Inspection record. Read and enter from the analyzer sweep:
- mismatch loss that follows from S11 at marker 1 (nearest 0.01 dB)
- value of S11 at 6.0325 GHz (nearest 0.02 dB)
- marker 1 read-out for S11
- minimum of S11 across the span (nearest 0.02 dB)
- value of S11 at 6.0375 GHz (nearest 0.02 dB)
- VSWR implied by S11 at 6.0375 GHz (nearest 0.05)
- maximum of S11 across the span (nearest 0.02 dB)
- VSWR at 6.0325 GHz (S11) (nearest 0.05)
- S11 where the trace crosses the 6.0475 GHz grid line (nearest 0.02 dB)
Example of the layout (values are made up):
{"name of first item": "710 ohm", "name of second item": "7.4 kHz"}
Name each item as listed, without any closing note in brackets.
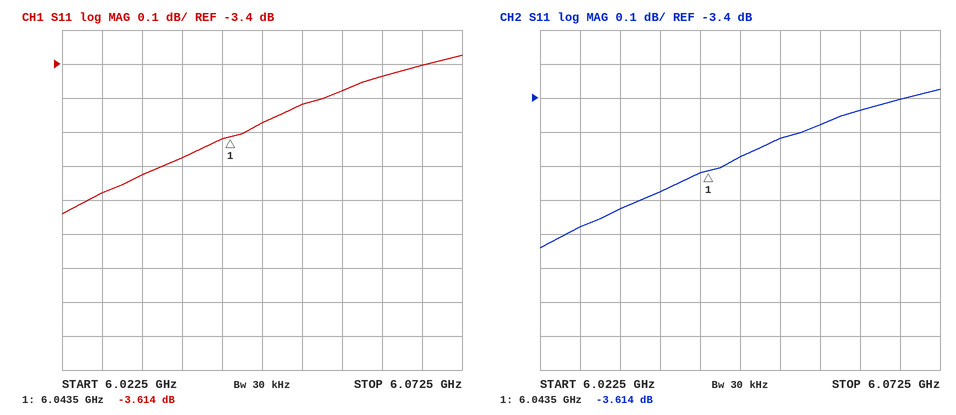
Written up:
{"mismatch loss that follows from S11 at marker 1": "2.48 dB", "value of S11 at 6.0325 GHz": "-3.72 dB", "marker 1 read-out for S11": "-3.614 dB", "minimum of S11 across the span": "-3.84 dB", "value of S11 at 6.0375 GHz": "-3.68 dB", "VSWR implied by S11 at 6.0375 GHz": "4.80", "maximum of S11 across the span": "-3.38 dB", "VSWR at 6.0325 GHz (S11)": "4.75", "S11 where the trace crosses the 6.0475 GHz grid line": "-3.58 dB"}
